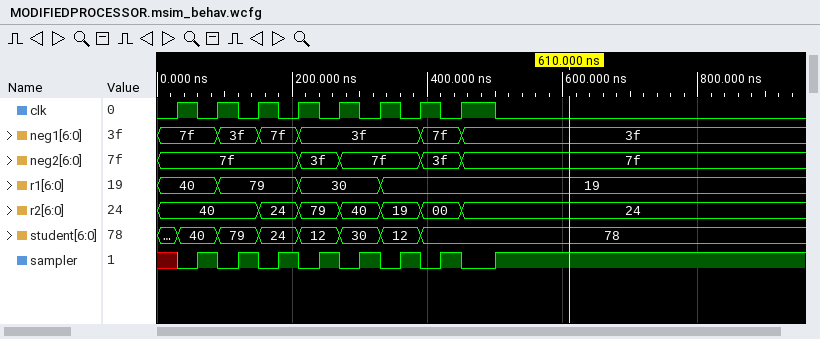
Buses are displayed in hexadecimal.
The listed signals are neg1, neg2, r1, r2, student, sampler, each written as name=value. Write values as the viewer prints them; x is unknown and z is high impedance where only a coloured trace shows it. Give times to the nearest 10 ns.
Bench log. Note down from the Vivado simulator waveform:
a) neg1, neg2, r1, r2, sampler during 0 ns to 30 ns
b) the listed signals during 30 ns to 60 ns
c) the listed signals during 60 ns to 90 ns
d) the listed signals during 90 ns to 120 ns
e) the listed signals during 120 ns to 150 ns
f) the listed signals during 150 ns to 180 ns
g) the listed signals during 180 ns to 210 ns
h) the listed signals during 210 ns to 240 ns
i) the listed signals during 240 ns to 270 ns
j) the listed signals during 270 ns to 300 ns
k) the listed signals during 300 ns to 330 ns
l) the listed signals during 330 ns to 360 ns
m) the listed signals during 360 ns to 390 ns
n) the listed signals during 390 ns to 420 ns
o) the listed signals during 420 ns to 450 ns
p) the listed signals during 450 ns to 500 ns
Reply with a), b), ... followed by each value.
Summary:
a) neg1=7f, neg2=7f, r1=40, r2=40, sampler=x
b) neg1=7f, neg2=7f, r1=40, r2=40, student=40, sampler=0
c) neg1=7f, neg2=7f, r1=40, r2=40, student=40, sampler=1
d) neg1=3f, neg2=7f, r1=79, r2=40, student=79, sampler=0
e) neg1=3f, neg2=7f, r1=79, r2=40, student=79, sampler=1
f) neg1=7f, neg2=7f, r1=79, r2=24, student=24, sampler=0
g) neg1=7f, neg2=7f, r1=79, r2=24, student=24, sampler=1
h) neg1=3f, neg2=3f, r1=30, r2=79, student=12, sampler=0
i) neg1=3f, neg2=3f, r1=30, r2=79, student=12, sampler=1
j) neg1=3f, neg2=7f, r1=30, r2=40, student=30, sampler=0
k) neg1=3f, neg2=7f, r1=30, r2=40, student=30, sampler=1
l) neg1=3f, neg2=7f, r1=19, r2=19, student=12, sampler=0
m) neg1=3f, neg2=7f, r1=19, r2=19, student=12, sampler=1
n) neg1=7f, neg2=3f, r1=19, r2=00, student=78, sampler=0
o) neg1=7f, neg2=3f, r1=19, r2=00, student=78, sampler=1
p) neg1=3f, neg2=7f, r1=19, r2=24, student=78, sampler=0
